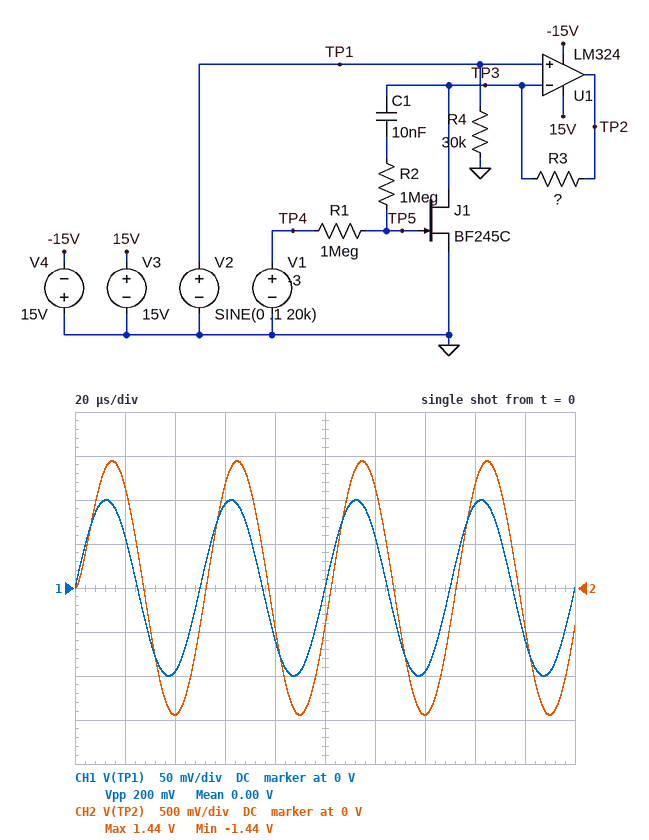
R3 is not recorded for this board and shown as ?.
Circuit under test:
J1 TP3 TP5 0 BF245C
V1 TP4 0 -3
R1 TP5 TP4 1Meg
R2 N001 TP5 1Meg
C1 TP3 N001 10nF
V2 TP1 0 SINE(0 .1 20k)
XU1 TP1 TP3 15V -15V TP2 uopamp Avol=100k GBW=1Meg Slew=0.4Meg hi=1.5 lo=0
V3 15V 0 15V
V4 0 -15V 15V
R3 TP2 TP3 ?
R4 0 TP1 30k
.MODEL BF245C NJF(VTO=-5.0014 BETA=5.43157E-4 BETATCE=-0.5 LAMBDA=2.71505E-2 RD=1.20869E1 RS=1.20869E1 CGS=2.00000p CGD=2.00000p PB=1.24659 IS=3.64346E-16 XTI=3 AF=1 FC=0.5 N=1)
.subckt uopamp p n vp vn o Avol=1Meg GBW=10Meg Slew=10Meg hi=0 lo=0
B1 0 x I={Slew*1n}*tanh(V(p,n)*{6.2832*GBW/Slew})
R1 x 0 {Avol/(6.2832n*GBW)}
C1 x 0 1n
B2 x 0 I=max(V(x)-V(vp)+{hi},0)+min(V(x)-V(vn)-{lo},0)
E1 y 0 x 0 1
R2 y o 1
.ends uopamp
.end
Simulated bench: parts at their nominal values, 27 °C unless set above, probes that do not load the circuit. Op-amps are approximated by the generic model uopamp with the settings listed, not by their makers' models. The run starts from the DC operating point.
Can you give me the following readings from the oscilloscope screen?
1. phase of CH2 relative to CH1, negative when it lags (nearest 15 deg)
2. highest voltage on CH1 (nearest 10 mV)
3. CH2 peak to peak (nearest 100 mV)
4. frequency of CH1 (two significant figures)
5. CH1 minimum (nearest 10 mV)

-15 deg
100 mV
2.9 V
20 kHz
-100 mV
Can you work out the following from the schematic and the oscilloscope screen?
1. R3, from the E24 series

6.8 kΩ
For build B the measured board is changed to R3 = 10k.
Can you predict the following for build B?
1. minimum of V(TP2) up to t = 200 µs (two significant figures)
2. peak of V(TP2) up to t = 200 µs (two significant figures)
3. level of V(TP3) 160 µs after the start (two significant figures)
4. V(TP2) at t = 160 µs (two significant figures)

-2.0 V
2.0 V
65 mV
1.4 V
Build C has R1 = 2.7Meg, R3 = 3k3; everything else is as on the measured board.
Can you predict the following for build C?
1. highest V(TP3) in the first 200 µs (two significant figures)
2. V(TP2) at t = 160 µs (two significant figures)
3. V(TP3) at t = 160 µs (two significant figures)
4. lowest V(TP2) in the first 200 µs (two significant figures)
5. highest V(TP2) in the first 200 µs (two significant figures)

99 mV
690 mV
88 mV
-770 mV
780 mV
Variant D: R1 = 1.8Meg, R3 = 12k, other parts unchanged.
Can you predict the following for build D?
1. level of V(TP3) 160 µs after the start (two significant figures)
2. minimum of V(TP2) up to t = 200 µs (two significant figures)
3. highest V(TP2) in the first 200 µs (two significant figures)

56 mV
-2.2 V
2.3 V
